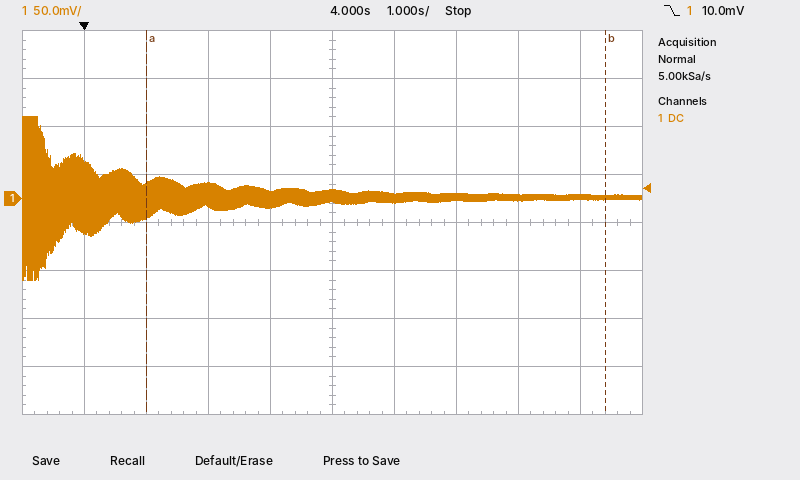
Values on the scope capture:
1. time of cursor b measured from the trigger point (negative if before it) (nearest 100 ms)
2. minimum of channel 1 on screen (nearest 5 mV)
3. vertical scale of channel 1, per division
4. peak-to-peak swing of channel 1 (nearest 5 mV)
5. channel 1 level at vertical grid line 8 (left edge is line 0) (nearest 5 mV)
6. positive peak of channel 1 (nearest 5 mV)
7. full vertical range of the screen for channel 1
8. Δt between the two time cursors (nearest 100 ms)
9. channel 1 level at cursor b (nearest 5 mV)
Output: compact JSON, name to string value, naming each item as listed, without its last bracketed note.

{"time of cursor b measured from the trigger point (negative if before it)": "+8.4 s", "minimum of channel 1 on screen": "-85 mV", "vertical scale of channel 1, per division": "50 mV", "peak-to-peak swing of channel 1": "170 mV", "channel 1 level at vertical grid line 8 (left edge is line 0)": "0 mV", "positive peak of channel 1": "85 mV", "full vertical range of the screen for channel 1": "400 mV", "Δt between the two time cursors": "7.4 s", "channel 1 level at cursor b": "0 mV"}
